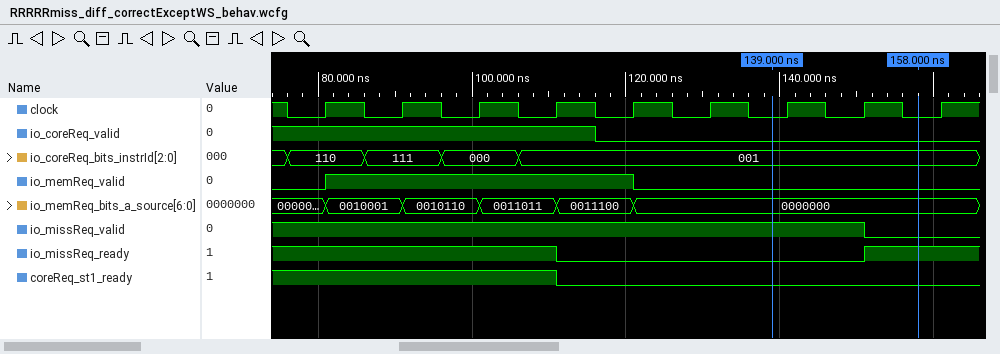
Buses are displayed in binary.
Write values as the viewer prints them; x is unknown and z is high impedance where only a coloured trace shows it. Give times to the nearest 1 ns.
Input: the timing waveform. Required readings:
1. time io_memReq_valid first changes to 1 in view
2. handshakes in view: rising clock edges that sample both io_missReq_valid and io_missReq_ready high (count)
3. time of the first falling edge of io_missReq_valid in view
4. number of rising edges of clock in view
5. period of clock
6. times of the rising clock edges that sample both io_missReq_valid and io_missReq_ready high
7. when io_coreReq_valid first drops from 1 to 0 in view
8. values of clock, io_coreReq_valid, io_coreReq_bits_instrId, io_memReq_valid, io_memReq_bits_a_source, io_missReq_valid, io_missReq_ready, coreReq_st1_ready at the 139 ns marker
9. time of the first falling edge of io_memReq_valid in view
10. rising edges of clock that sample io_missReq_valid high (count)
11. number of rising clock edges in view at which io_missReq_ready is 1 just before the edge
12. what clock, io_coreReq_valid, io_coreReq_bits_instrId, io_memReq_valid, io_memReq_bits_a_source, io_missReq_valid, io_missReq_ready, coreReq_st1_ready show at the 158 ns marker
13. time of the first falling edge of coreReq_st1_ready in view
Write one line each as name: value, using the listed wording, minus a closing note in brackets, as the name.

time io_memReq_valid first changes to 1 in view: 81 ns
handshakes in view: rising clock edges that sample both io_missReq_valid and io_missReq_ready high: 4
time of the first falling edge of io_missReq_valid in view: 151 ns
number of rising edges of clock in view: 9
period of clock: 10 ns
times of the rising clock edges that sample both io_missReq_valid and io_missReq_ready high: 81 ns, 91 ns, 101 ns, 111 ns
when io_coreReq_valid first drops from 1 to 0 in view: 116 ns
values of clock, io_coreReq_valid, io_coreReq_bits_instrId, io_memReq_valid, io_memReq_bits_a_source, io_missReq_valid, io_missReq_ready, coreReq_st1_ready at the 139 ns marker: clock=0, io_coreReq_valid=0, io_coreReq_bits_instrId=001, io_memReq_valid=0, io_memReq_bits_a_source=0000000, io_missReq_valid=1, io_missReq_ready=0, coreReq_st1_ready=0
time of the first falling edge of io_memReq_valid in view: 121 ns
rising edges of clock that sample io_missReq_valid high: 8
number of rising clock edges in view at which io_missReq_ready is 1 just before the edge: 5
what clock, io_coreReq_valid, io_coreReq_bits_instrId, io_memReq_valid, io_memReq_bits_a_source, io_missReq_valid, io_missReq_ready, coreReq_st1_ready show at the 158 ns marker: clock=0, io_coreReq_valid=0, io_coreReq_bits_instrId=001, io_memReq_valid=0, io_memReq_bits_a_source=0000000, io_missReq_valid=0, io_missReq_ready=1, coreReq_st1_ready=0
time of the first falling edge of coreReq_st1_ready in view: 111 ns
